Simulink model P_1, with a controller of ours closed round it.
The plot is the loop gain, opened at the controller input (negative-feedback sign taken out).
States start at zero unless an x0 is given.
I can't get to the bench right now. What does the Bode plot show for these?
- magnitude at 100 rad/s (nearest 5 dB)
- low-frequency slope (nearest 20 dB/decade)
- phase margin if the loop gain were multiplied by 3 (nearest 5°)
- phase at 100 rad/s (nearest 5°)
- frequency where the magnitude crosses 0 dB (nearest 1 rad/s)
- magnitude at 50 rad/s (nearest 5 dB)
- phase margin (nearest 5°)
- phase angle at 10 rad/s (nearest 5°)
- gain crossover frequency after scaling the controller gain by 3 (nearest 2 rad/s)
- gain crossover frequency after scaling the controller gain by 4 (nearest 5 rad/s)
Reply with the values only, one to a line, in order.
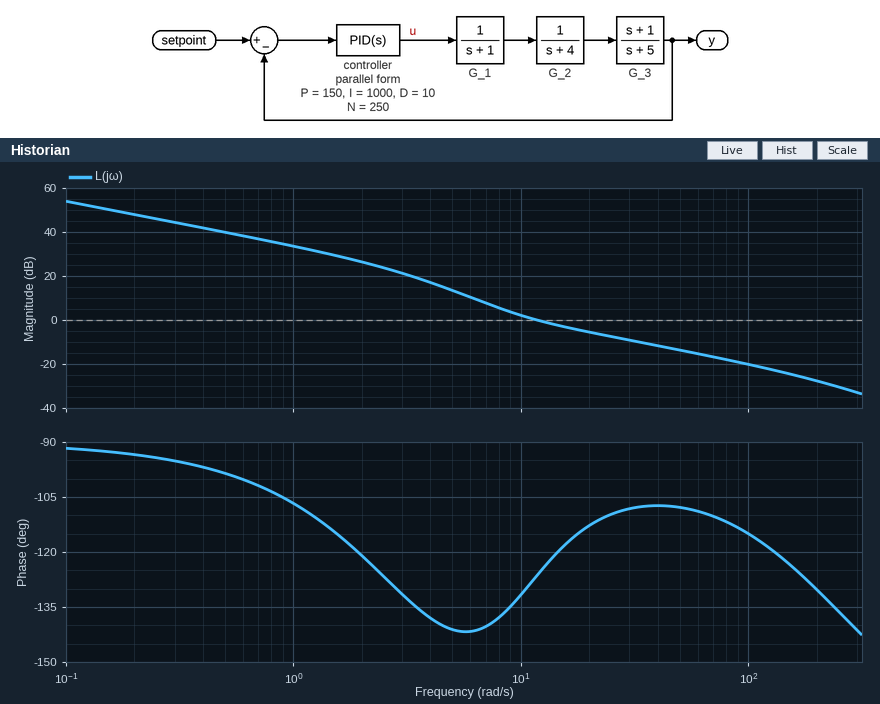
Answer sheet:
-20 dB
-20 dB/decade
70°
-115°
12 rad/s
-15 dB
55°
-130°
32 rad/s
40 rad/s
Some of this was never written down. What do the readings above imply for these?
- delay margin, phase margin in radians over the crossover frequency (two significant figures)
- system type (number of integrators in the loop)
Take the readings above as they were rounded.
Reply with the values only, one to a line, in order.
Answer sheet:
0.080 s
1
